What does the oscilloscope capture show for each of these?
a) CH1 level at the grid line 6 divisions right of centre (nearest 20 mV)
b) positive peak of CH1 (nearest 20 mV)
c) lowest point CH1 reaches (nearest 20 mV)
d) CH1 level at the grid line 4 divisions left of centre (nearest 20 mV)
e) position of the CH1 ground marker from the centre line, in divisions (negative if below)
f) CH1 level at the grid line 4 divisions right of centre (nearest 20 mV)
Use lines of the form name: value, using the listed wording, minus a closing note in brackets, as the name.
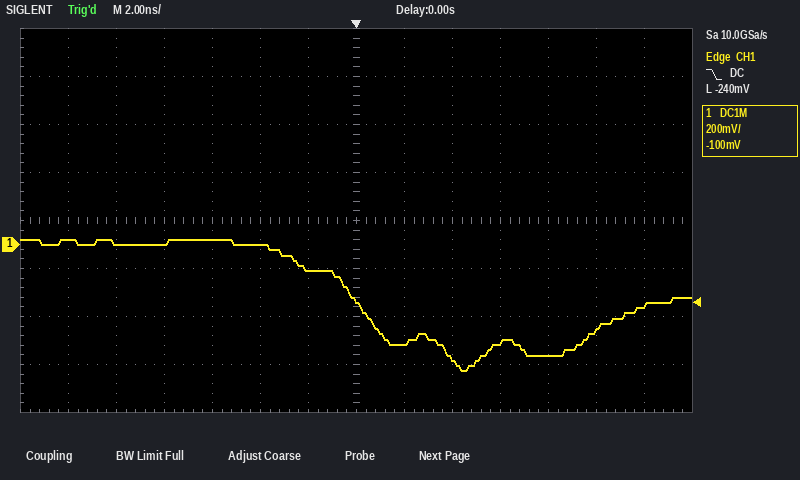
CH1 level at the grid line 6 divisions right of centre: -260 mV
positive peak of CH1: 20 mV
lowest point CH1 reaches: -520 mV
CH1 level at the grid line 4 divisions left of centre: 0 mV
position of the CH1 ground marker from the centre line, in divisions: -0.5 div
CH1 level at the grid line 4 divisions right of centre: -460 mV
